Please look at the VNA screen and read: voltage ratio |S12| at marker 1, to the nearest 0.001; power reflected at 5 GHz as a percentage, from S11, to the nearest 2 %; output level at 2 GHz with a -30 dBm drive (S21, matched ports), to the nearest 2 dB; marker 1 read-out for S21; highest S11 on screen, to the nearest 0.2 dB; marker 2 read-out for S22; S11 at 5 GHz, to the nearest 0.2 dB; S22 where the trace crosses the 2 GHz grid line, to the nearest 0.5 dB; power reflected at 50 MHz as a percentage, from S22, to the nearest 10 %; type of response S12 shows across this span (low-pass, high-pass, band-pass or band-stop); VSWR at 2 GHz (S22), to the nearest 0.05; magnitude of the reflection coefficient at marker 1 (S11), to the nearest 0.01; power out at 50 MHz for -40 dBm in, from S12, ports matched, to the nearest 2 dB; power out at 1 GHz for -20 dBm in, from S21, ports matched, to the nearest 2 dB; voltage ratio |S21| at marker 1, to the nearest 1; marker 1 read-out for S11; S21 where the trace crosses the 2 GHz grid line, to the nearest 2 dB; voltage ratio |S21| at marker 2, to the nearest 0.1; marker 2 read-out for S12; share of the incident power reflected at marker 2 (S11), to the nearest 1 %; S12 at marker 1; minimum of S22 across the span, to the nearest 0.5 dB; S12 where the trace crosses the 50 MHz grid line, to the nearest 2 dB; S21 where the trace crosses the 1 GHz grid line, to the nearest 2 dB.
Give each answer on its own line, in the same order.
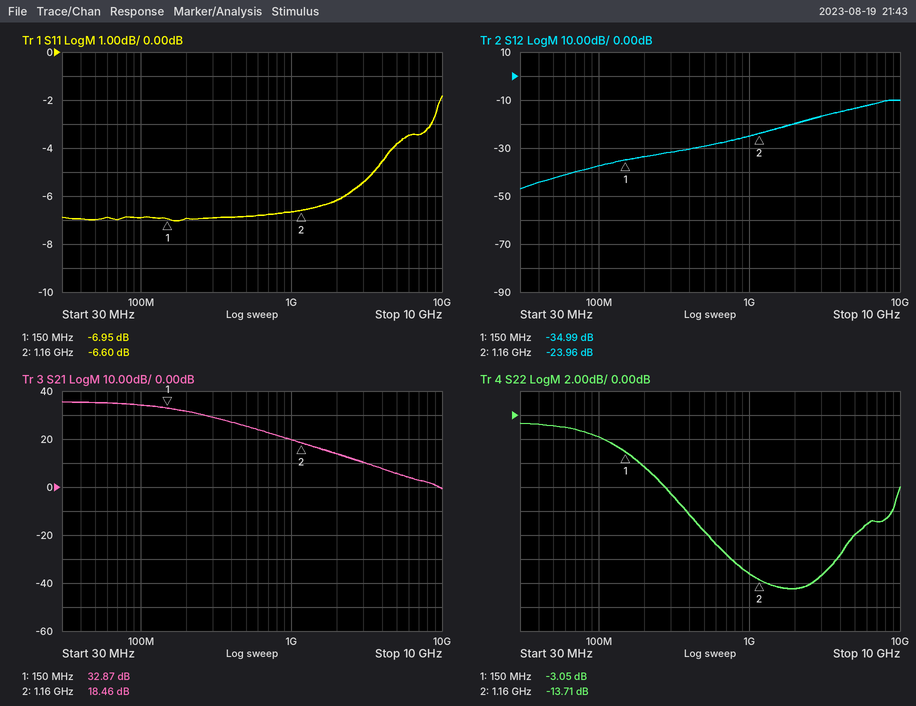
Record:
0.018
42 %
-16 dBm
32.87 dB
-1.8 dB
-13.71 dB
-3.8 dB
-14.5 dB
80 %
high-pass
1.45
0.45
-82 dBm
0 dBm
44
-6.95 dB
14 dB
8.4
-23.96 dB
22 %
-34.99 dB
-14.5 dB
-42 dB
20 dB
